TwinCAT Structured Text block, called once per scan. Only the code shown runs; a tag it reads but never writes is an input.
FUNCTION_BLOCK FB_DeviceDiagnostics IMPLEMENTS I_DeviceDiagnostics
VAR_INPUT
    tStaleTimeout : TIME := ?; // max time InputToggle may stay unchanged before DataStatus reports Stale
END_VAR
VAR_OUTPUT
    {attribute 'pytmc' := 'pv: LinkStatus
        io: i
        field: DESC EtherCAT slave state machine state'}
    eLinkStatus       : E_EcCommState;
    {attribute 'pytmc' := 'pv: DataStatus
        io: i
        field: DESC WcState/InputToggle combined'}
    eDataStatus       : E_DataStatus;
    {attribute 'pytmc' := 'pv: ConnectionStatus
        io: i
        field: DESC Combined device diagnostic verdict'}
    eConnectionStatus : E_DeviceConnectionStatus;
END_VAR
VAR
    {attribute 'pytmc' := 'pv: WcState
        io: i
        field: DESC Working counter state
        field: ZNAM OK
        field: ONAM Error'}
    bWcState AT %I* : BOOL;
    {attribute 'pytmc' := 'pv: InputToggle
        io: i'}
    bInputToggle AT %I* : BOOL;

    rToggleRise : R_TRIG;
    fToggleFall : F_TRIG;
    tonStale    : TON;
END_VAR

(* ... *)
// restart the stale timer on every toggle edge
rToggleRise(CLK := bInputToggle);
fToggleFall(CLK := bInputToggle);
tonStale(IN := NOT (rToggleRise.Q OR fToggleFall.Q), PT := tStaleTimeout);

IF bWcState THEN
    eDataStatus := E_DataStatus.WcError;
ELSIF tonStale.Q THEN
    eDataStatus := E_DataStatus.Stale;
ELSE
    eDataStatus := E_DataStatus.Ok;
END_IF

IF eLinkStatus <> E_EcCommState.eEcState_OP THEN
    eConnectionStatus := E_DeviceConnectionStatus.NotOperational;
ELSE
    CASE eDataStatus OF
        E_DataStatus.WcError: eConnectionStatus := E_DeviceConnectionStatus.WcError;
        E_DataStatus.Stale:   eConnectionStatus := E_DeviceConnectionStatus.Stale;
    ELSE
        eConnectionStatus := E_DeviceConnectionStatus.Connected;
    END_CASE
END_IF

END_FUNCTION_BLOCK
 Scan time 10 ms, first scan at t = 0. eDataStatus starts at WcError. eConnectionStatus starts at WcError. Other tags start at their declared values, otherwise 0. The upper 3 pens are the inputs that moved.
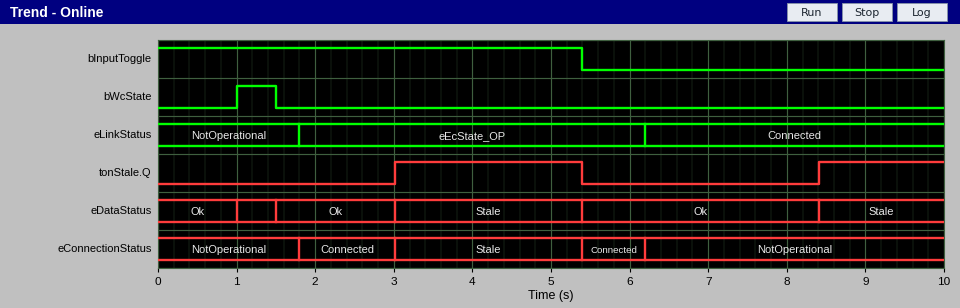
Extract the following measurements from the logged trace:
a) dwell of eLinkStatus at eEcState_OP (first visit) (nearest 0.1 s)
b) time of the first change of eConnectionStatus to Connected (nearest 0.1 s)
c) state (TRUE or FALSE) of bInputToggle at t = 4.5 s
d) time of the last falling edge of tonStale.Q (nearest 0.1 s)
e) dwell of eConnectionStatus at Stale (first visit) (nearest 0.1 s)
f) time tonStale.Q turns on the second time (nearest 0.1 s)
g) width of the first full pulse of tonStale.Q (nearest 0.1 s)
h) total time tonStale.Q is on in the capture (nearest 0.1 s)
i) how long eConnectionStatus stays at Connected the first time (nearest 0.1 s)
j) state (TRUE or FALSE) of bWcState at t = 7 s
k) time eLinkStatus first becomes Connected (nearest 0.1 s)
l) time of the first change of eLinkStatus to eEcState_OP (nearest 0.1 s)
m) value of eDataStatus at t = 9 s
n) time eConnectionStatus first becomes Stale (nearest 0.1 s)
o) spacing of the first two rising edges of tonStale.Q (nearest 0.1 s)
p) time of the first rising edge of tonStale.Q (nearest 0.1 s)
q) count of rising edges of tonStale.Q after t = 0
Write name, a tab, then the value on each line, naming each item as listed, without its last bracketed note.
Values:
dwell of eLinkStatus at eEcState_OP (first visit)	4.4 s
time of the first change of eConnectionStatus to Connected	1.8 s
state (TRUE or FALSE) of bInputToggle at t = 4.5 s	TRUE
time of the last falling edge of tonStale.Q	5.4 s
dwell of eConnectionStatus at Stale (first visit)	2.4 s
time tonStale.Q turns on the second time	8.4 s
width of the first full pulse of tonStale.Q	2.4 s
total time tonStale.Q is on in the capture	4.0 s
how long eConnectionStatus stays at Connected the first time	1.2 s
state (TRUE or FALSE) of bWcState at t = 7 s	FALSE
time eLinkStatus first becomes Connected	6.2 s
time of the first change of eLinkStatus to eEcState_OP	1.8 s
value of eDataStatus at t = 9 s	Stale
time eConnectionStatus first becomes Stale	3.0 s
spacing of the first two rising edges of tonStale.Q	5.4 s
time of the first rising edge of tonStale.Q	3.0 s
count of rising edges of tonStale.Q after t = 0	2
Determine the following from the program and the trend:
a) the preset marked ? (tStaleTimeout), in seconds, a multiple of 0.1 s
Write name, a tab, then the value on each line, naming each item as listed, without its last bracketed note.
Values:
the preset marked ? (tStaleTimeout), in seconds, a multiple of 0.1 s	3.0 s
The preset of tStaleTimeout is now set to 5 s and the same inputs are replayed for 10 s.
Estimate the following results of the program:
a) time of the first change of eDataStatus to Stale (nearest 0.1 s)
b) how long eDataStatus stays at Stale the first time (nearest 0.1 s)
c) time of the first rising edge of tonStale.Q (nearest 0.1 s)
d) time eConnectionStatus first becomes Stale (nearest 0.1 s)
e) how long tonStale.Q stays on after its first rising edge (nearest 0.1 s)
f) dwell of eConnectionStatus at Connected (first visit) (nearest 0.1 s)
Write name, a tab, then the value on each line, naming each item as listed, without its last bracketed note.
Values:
time of the first change of eDataStatus to Stale	5.0 s
how long eDataStatus stays at Stale the first time	0.4 s
time of the first rising edge of tonStale.Q	5.0 s
time eConnectionStatus first becomes Stale	5.0 s
how long tonStale.Q stays on after its first rising edge	0.4 s
dwell of eConnectionStatus at Connected (first visit)	3.2 s
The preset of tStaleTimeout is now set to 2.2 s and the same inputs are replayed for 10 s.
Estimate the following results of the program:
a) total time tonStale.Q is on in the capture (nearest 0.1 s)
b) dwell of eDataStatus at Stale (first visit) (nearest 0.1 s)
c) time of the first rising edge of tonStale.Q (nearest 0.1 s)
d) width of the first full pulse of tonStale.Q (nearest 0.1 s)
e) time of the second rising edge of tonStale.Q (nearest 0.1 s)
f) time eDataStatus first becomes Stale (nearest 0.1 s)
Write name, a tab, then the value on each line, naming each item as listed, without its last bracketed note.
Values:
total time tonStale.Q is on in the capture	5.6 s
dwell of eDataStatus at Stale (first visit)	3.2 s
time of the first rising edge of tonStale.Q	2.2 s
width of the first full pulse of tonStale.Q	3.2 s
time of the second rising edge of tonStale.Q	7.6 s
time eDataStatus first becomes Stale	2.2 s
